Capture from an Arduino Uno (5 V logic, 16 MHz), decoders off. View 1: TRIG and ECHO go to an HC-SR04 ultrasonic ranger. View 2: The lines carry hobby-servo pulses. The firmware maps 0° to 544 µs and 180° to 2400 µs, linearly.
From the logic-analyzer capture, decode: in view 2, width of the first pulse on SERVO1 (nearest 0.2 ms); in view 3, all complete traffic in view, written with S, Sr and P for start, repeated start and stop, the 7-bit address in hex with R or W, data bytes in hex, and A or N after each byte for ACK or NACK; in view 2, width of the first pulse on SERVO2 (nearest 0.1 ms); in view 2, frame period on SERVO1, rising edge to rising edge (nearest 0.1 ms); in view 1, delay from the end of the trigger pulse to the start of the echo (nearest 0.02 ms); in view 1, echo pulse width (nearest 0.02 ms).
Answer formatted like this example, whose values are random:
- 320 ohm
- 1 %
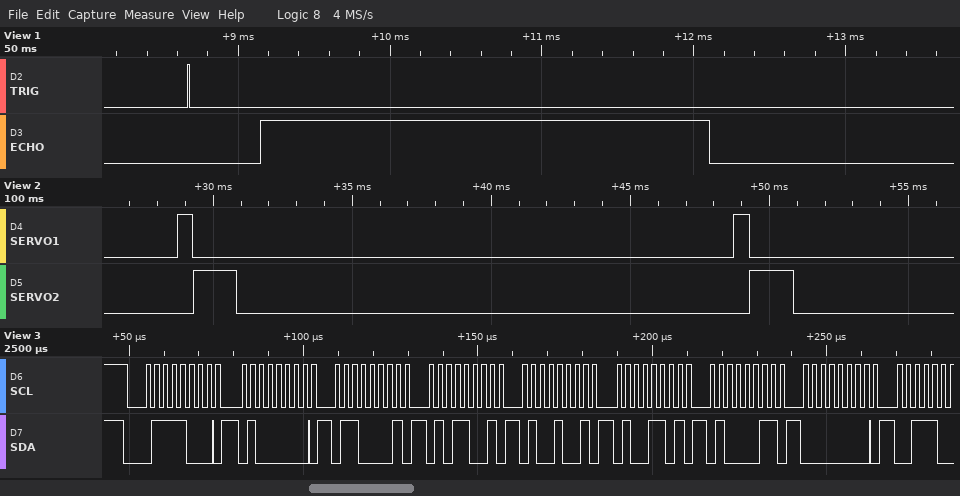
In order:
- 0.6 ms
- S 3CW A 40 A 61 A 59 A 49 A 4D A 43 A 00 A
- 1.6 ms
- 20.0 ms
- 0.46 ms
- 2.96 ms
